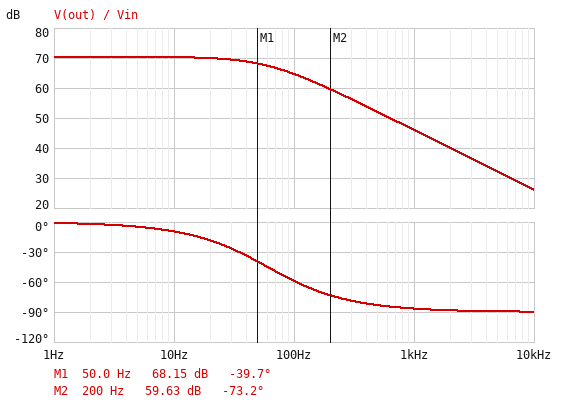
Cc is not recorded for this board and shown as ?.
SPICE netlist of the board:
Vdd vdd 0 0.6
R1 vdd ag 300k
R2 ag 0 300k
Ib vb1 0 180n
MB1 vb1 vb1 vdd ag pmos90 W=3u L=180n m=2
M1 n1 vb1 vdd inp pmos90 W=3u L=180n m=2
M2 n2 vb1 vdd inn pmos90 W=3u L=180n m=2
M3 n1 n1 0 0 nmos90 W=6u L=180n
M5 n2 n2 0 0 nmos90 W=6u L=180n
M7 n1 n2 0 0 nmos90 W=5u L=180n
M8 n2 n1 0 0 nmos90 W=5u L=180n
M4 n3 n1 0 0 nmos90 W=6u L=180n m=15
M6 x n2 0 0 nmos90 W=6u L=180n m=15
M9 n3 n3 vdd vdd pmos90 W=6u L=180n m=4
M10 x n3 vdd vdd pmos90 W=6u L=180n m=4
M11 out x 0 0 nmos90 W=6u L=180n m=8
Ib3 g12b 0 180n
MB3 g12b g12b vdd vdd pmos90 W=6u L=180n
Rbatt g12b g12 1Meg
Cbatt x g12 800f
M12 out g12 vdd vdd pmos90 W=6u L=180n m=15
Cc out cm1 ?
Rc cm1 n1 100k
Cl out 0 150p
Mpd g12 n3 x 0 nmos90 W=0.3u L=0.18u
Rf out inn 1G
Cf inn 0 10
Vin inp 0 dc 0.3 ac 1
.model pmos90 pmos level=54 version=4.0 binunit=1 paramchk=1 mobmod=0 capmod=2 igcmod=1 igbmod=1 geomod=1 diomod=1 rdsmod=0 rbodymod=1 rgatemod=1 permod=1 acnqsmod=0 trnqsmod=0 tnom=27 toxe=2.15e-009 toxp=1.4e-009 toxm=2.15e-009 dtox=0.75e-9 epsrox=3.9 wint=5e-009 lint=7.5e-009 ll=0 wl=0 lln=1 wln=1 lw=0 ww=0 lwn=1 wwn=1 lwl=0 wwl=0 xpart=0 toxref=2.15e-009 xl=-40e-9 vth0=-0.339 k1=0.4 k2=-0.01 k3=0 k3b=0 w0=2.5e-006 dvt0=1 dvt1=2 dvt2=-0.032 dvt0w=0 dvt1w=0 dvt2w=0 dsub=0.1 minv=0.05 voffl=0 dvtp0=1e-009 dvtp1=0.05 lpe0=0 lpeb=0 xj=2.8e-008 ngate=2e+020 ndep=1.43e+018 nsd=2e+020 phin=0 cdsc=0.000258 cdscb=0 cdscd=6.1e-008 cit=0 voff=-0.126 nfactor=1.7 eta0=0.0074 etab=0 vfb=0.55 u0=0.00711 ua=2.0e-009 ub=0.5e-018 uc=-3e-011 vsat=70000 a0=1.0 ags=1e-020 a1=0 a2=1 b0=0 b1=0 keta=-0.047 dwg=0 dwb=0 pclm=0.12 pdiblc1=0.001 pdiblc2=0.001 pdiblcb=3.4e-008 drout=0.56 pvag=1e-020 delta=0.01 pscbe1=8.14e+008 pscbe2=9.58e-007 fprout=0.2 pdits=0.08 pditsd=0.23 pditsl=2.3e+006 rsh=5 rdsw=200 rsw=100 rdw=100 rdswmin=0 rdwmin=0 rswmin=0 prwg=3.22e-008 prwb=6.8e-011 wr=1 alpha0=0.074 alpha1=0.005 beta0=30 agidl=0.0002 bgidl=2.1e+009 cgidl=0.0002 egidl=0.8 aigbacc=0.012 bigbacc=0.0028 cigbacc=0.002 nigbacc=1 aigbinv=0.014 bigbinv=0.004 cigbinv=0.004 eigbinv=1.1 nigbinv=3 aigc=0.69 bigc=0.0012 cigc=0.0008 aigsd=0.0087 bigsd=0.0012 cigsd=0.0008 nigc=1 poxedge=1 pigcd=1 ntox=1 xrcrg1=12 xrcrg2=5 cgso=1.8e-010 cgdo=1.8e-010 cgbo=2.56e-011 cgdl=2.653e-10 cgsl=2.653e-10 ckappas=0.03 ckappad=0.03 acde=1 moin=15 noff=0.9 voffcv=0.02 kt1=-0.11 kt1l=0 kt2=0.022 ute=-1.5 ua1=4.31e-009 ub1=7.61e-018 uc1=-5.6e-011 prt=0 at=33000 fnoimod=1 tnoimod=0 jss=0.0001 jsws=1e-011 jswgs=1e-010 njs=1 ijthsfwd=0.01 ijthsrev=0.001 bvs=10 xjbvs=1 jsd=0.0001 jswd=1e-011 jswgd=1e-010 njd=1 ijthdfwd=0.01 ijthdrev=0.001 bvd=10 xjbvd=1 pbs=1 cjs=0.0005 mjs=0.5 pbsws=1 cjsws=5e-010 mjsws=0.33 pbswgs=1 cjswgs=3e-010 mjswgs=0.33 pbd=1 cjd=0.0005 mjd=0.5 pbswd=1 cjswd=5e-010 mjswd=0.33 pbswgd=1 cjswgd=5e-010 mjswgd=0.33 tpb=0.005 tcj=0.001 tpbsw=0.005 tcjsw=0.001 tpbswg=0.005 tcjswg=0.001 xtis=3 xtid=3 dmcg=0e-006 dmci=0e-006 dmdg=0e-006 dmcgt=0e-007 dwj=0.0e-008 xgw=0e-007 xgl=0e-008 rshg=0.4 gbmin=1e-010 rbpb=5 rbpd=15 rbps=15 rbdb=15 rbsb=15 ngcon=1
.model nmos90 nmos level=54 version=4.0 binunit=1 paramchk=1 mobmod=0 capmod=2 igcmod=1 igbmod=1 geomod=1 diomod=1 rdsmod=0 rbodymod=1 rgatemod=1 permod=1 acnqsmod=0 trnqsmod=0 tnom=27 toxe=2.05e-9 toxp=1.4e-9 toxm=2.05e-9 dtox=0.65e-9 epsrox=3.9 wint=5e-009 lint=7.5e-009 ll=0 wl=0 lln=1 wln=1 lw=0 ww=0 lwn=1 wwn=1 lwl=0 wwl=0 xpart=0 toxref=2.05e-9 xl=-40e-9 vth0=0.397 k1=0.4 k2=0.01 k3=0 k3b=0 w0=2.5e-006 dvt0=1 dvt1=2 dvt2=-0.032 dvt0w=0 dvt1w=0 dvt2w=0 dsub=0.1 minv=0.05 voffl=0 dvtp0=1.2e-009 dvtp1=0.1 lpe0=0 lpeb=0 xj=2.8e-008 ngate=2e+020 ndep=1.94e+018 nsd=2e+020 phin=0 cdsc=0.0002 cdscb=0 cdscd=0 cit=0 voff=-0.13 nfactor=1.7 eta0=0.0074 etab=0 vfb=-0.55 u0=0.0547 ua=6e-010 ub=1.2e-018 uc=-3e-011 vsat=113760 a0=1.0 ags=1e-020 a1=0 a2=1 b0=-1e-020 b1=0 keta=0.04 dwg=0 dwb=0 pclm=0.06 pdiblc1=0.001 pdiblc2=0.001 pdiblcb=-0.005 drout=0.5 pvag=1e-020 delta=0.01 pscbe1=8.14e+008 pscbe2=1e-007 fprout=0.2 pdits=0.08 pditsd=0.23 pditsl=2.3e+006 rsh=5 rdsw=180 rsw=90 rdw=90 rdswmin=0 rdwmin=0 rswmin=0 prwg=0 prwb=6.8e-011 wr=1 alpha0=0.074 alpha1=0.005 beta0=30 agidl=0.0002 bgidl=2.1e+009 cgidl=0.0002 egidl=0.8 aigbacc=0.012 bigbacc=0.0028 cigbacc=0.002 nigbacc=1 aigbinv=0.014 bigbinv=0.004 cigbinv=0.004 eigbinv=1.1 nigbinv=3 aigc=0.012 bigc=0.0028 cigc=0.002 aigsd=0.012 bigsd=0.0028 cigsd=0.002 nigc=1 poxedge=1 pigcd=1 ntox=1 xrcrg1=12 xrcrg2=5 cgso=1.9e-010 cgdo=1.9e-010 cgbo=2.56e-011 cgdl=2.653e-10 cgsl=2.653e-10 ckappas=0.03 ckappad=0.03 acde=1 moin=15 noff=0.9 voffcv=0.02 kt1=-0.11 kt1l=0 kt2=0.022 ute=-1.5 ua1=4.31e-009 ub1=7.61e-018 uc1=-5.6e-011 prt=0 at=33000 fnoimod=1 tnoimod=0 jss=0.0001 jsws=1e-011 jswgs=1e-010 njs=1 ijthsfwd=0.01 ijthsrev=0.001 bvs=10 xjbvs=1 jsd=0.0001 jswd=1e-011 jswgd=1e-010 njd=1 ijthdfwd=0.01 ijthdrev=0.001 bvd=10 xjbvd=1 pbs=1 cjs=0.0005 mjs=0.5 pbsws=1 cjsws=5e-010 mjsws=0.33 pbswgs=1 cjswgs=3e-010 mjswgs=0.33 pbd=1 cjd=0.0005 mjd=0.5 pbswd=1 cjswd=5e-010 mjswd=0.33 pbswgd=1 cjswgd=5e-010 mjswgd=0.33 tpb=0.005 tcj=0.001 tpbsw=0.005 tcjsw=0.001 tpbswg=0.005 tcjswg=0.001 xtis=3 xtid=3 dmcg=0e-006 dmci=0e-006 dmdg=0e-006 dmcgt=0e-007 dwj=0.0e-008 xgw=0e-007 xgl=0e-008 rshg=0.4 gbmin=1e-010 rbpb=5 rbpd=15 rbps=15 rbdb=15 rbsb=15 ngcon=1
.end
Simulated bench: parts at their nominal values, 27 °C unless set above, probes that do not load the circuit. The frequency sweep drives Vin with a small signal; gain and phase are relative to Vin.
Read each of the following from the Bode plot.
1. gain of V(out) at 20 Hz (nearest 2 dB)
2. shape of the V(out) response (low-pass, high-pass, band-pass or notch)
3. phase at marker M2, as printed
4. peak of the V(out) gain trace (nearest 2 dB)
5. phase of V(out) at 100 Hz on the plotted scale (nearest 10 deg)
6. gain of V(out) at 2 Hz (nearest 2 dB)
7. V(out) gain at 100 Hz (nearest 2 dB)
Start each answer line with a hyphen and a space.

- 70 dB
- low-pass
- -73.2 deg
- 70 dB
- -60 deg
- 70 dB
- 64 dB
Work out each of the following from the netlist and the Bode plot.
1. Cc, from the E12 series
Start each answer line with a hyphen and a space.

- 1 pF
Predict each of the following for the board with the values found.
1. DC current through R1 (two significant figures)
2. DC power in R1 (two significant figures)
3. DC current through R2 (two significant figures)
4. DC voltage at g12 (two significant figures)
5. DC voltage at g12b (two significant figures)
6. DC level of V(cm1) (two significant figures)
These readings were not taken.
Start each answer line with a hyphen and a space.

- 1.0 µA
- 300 nW
- 1.0 µA
- 400 mV
- 410 mV
- 130 mV
